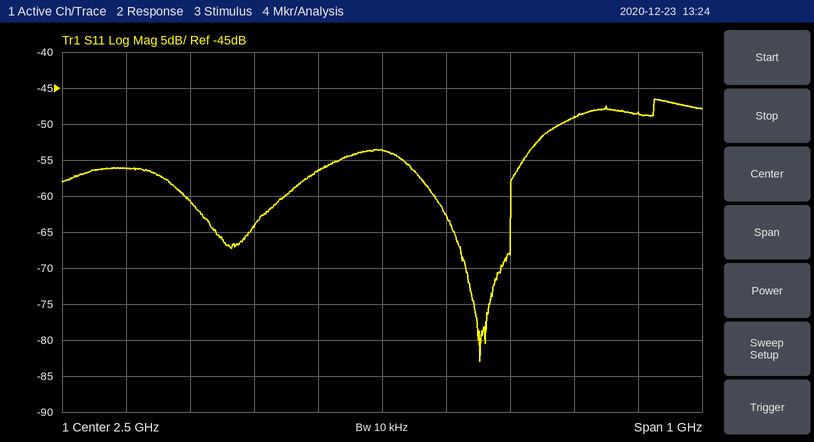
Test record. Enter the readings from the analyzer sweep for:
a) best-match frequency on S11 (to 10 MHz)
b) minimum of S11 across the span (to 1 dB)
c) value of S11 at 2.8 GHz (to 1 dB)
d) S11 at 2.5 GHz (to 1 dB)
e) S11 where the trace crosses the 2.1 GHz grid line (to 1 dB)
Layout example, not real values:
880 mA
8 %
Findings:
2.65 GHz
-83 dB
-49 dB
-54 dB
-56 dB
